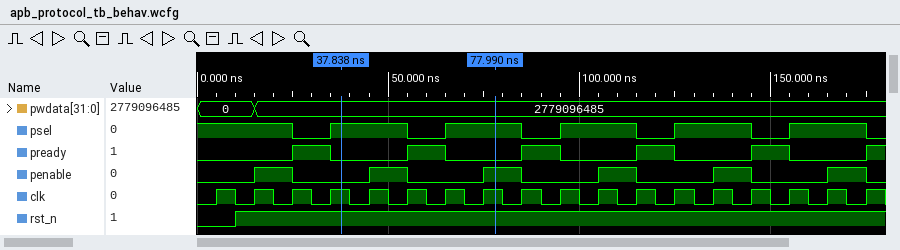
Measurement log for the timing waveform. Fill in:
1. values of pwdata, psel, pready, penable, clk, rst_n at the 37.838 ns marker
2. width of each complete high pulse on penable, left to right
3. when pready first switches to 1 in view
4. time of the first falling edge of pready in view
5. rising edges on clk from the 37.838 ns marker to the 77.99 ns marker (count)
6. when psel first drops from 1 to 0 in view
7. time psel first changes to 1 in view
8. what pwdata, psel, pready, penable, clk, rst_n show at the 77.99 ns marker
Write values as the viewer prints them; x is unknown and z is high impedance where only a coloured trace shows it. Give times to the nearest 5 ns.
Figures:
pwdata=2779096485, psel=1, pready=0, penable=0, clk=1, rst_n=1
10 ns, 10 ns, 10 ns, 10 ns, 10 ns, 10 ns
25 ns
35 ns
4
25 ns
35 ns
pwdata=2779096485, psel=1, pready=0, penable=1, clk=1, rst_n=1
